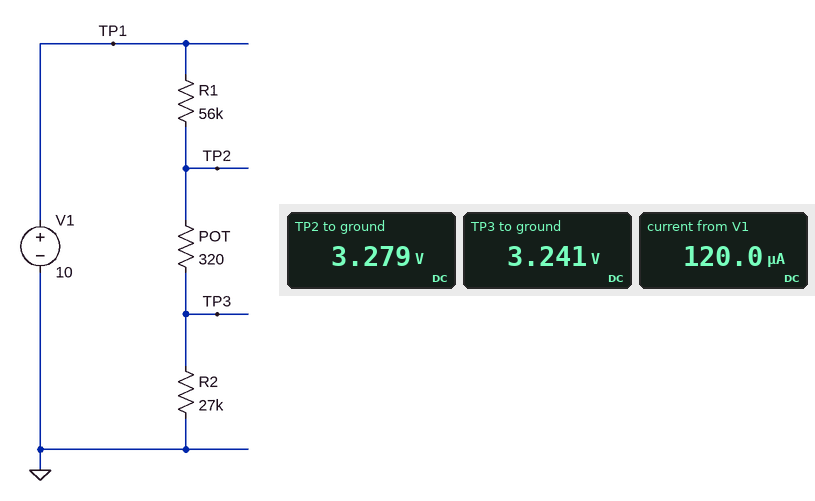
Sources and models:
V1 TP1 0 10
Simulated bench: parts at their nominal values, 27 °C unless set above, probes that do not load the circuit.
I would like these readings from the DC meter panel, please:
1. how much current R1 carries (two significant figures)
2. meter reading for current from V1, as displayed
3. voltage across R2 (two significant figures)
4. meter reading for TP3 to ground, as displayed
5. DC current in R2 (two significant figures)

120 µA
120.0 µA
3.2 V
3.241 V
120 µA
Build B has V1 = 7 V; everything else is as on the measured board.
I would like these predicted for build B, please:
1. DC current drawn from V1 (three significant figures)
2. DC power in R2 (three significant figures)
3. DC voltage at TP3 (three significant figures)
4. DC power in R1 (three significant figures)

84.0 µA
191 µW
2.27 V
395 µW
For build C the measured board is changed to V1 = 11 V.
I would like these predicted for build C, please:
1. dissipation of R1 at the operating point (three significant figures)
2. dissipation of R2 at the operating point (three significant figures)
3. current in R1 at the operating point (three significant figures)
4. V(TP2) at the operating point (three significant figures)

976 µW
471 µW
132 µA
3.61 V
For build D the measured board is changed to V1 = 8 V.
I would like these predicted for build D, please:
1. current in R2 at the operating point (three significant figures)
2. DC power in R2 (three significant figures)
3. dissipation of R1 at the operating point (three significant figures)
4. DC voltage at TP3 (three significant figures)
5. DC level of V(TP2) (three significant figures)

96.0 µA
249 µW
516 µW
2.59 V
2.62 V
